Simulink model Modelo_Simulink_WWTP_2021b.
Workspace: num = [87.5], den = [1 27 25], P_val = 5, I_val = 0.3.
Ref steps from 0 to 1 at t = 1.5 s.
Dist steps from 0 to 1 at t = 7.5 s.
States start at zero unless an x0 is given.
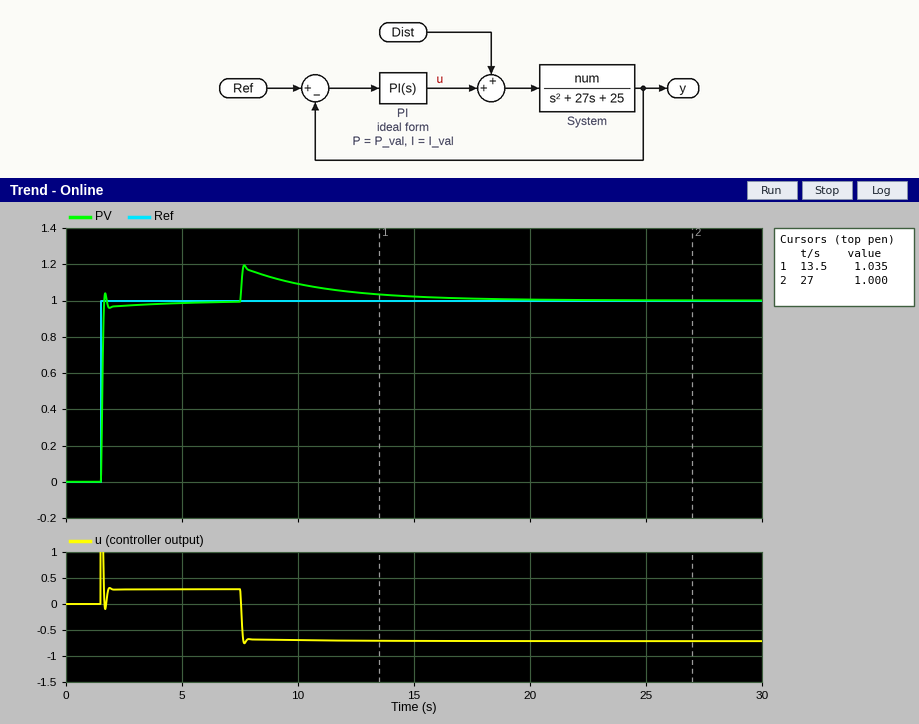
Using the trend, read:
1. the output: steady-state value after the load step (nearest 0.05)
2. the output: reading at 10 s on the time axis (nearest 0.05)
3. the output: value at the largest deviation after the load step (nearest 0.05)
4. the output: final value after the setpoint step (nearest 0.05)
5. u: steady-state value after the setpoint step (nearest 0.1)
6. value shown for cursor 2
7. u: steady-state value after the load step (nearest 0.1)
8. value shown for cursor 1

1.00
1.10
1.20
1.00
0.3
1.000
-0.7
1.035
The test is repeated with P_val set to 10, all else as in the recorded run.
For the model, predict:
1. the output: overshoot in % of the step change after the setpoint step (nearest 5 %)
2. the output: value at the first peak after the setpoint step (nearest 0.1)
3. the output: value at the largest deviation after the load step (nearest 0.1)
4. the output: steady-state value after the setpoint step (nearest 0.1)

20 %
1.2
1.1
1.0
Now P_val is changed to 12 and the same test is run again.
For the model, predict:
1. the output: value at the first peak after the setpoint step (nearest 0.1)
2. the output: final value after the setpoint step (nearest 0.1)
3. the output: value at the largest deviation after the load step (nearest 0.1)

1.2
1.0
1.1
